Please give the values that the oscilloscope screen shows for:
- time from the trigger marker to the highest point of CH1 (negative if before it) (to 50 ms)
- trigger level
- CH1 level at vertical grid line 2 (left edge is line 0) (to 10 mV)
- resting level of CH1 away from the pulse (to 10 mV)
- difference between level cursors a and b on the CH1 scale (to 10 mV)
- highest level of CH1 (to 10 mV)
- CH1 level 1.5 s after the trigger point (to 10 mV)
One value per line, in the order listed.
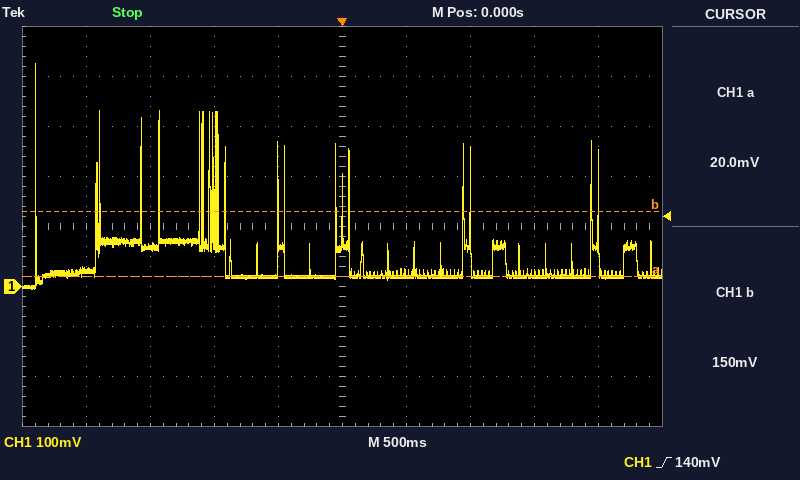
-2.40 s
140 mV
80 mV
20 mV
130 mV
450 mV
30 mV
